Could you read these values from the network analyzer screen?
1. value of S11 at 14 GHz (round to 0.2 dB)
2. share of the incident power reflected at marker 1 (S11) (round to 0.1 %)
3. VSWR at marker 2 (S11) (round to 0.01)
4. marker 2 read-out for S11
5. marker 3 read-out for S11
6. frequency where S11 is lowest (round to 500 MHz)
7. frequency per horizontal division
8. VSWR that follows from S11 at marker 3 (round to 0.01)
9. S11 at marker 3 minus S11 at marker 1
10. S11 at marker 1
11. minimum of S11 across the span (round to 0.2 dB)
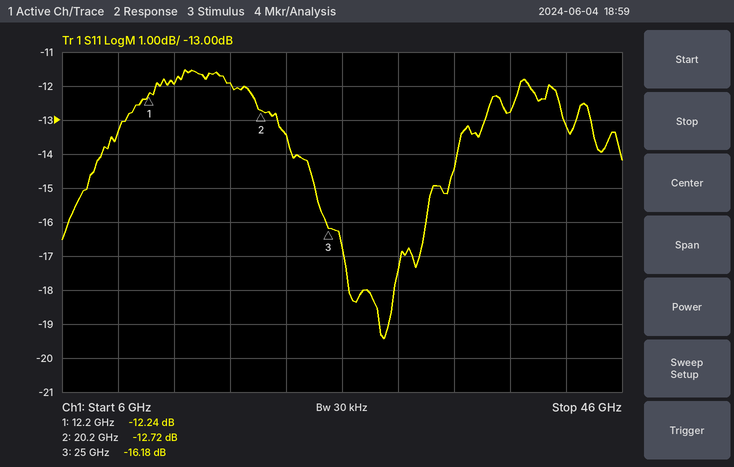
-12.0 dB
6.0 %
1.60
-12.72 dB
-16.18 dB
29.0 GHz
4 GHz
1.37
-3.94 dB
-12.24 dB
-19.4 dB
